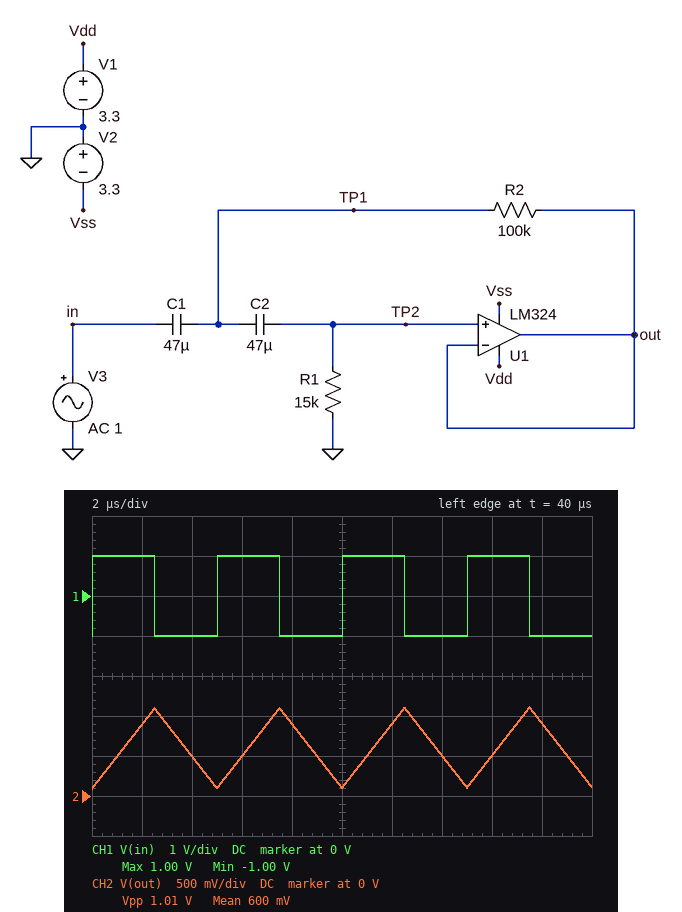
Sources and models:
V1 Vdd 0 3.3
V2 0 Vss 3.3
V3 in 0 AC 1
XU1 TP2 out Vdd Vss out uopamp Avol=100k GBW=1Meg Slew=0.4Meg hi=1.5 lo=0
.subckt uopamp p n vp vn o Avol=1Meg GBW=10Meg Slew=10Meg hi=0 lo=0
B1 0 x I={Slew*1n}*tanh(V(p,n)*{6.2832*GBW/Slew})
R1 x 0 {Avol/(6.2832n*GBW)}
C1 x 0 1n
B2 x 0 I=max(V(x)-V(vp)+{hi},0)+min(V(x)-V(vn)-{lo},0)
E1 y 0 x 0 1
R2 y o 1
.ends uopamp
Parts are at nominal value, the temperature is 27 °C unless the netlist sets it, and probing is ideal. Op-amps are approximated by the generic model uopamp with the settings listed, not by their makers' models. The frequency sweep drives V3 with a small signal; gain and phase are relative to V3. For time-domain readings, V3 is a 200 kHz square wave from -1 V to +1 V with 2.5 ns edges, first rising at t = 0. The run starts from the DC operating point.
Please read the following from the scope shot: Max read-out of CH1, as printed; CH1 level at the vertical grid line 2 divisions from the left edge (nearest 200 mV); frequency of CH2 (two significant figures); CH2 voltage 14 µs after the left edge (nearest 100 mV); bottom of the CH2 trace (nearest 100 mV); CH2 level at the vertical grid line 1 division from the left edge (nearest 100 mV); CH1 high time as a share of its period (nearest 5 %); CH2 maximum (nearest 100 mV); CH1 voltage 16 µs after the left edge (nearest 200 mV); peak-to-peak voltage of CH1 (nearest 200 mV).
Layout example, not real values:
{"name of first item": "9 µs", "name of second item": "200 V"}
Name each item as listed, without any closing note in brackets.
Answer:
{"Max read-out of CH1, as printed": "1.00 V", "CH1 level at the vertical grid line 2 divisions from the left edge": "-1.0 V", "frequency of CH2": "200 kHz", "CH2 voltage 14 µs after the left edge": "500 mV", "bottom of the CH2 trace": "100 mV", "CH2 level at the vertical grid line 1 division from the left edge": "900 mV", "CH1 high time as a share of its period": "50 %", "CH2 maximum": "1.1 V", "CH1 voltage 16 µs after the left edge": "1.0 V", "peak-to-peak voltage of CH1": "2.0 V"}
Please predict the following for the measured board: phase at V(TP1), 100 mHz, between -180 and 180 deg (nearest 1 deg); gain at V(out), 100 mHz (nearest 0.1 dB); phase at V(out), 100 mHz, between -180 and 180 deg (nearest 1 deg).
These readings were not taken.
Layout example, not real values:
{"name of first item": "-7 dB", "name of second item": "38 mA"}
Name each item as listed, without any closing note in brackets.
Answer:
{"phase at V(TP1), 100 mHz, between -180 and 180 deg": "21 deg", "gain at V(out), 100 mHz": "-13.1 dB", "phase at V(out), 100 mHz, between -180 and 180 deg": "87 deg"}
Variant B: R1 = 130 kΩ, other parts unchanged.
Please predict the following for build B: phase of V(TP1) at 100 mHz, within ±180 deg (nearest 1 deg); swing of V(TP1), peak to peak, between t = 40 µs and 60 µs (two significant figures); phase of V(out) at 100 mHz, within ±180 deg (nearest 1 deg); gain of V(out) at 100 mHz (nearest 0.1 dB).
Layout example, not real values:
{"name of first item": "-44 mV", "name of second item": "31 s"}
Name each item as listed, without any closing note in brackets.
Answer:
{"phase of V(TP1) at 100 mHz, within ±180 deg": "15 deg", "swing of V(TP1), peak to peak, between t = 40 µs and 60 µs": "2.0 V", "phase of V(out) at 100 mHz, within ±180 deg": "30 deg", "gain of V(out) at 100 mHz": "-0.4 dB"}
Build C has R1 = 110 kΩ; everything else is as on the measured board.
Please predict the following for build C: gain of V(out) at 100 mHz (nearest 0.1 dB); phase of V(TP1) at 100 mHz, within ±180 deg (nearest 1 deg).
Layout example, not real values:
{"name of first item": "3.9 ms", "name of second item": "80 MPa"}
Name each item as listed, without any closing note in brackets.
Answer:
{"gain of V(out) at 100 mHz": "-0.7 dB", "phase of V(TP1) at 100 mHz, within ±180 deg": "17 deg"}
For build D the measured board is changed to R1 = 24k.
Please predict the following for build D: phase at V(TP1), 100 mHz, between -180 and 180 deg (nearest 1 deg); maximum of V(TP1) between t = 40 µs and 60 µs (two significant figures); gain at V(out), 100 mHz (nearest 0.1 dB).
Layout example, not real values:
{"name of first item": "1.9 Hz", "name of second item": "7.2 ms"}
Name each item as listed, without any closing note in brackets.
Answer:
{"phase at V(TP1), 100 mHz, between -180 and 180 deg": "25 deg", "maximum of V(TP1) between t = 40 µs and 60 µs": "2.0 V", "gain at V(out), 100 mHz": "-9.2 dB"}
